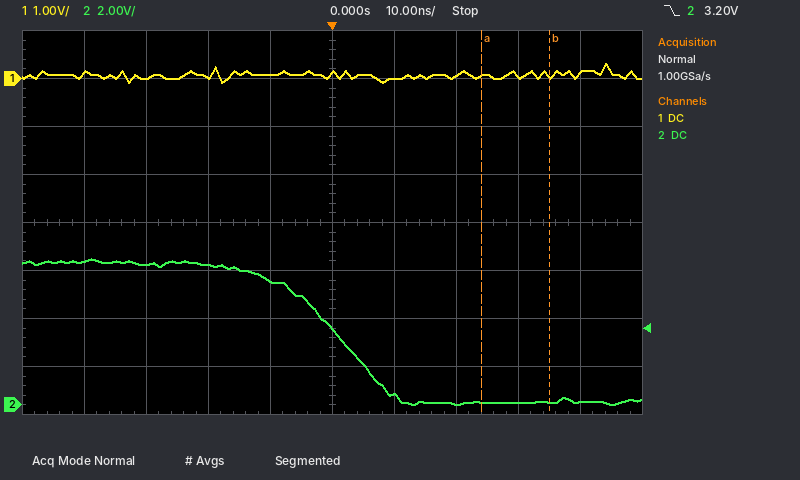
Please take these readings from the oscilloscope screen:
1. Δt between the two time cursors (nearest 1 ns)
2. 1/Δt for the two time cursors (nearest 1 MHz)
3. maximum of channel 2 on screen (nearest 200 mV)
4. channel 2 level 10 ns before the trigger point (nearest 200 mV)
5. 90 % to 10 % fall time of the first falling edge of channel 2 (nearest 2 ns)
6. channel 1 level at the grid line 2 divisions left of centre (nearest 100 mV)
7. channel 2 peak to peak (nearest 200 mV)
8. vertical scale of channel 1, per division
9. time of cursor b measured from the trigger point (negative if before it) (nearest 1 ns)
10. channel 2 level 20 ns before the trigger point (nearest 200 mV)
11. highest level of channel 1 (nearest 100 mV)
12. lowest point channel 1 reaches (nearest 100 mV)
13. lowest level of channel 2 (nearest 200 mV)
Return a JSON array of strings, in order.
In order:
["11 ns", "91 MHz", "6.0 V", "5.2 V", "20 ns", "0.0 V", "6.0 V", "1 V", "+35 ns", "5.8 V", "300 mV", "-100 mV", "0.0 V"]
